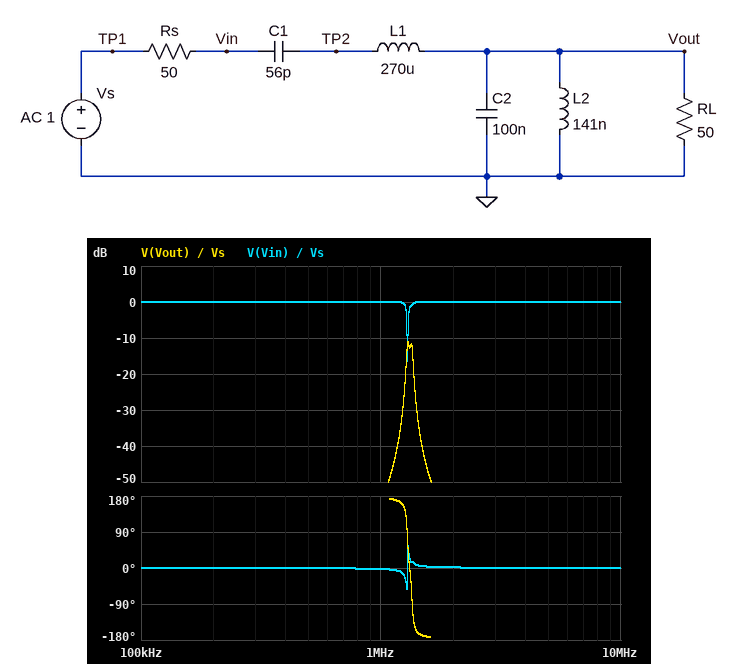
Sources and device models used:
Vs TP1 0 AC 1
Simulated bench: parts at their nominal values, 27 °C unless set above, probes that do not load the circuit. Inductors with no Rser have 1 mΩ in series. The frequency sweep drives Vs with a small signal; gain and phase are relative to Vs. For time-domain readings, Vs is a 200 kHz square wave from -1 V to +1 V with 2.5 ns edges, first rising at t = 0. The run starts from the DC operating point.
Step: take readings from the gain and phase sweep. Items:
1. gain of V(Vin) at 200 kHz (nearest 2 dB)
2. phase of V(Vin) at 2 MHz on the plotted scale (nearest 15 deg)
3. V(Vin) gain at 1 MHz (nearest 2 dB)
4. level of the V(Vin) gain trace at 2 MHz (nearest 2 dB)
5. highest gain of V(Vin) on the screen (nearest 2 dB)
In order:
0 dB
0 deg
0 dB
0 dB
0 dB
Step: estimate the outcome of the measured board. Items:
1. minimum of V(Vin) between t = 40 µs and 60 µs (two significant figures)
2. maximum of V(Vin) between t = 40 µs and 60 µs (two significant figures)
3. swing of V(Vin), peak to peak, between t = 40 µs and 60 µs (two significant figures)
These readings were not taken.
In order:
-1.0 V
1.0 V
2.1 V
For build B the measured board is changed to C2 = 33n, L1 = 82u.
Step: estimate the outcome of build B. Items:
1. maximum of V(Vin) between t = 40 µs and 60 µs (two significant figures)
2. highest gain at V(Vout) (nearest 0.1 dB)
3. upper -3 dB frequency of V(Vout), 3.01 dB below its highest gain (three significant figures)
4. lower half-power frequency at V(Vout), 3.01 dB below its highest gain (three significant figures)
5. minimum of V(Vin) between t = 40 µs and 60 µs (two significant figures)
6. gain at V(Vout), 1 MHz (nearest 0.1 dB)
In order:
1.1 V
-6.2 dB
2.41 MHz
2.27 MHz
-1.1 V
-66.6 dB
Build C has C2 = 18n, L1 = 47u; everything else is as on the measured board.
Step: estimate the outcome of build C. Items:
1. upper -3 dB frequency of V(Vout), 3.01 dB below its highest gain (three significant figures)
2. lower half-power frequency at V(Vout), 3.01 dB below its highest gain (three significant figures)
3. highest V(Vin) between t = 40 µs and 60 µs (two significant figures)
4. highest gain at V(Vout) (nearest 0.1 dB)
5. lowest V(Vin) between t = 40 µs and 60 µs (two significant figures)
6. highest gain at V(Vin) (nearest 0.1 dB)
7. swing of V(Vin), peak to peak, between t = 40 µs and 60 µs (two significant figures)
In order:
3.26 MHz
3.00 MHz
1.1 V
-6.5 dB
-1.1 V
0 dB
2.2 V
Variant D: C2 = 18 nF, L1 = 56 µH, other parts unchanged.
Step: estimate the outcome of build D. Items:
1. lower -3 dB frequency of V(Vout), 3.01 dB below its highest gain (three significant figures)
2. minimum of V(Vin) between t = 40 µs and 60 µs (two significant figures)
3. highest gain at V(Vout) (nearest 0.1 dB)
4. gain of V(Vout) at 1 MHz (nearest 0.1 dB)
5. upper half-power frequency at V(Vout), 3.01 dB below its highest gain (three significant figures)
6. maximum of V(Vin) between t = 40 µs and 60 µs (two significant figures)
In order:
2.78 MHz
-1.1 V
-12.6 dB
-68.1 dB
3.22 MHz
1.1 V
